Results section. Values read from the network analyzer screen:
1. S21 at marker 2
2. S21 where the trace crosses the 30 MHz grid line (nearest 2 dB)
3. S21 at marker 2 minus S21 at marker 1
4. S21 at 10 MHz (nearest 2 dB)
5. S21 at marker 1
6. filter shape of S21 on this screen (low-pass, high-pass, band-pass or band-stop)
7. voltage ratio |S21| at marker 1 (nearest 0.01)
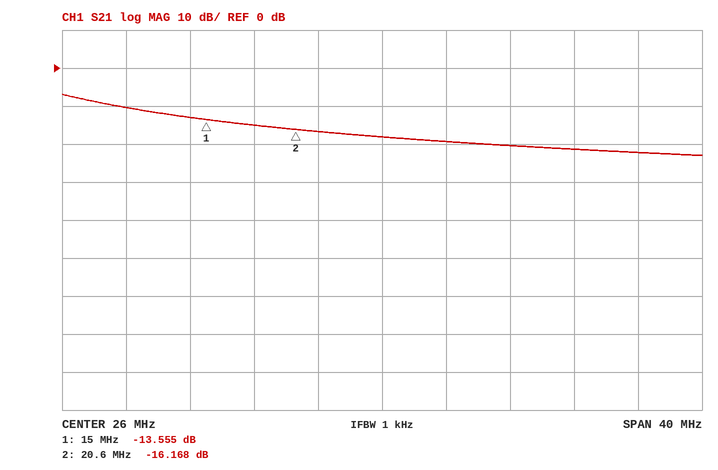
-16.168 dB
-20 dB
-2.613 dB
-10 dB
-13.555 dB
low-pass
0.21
